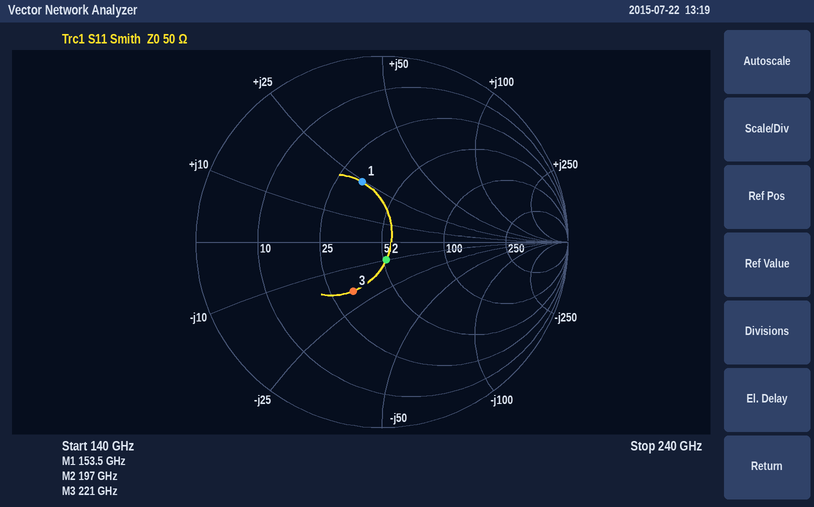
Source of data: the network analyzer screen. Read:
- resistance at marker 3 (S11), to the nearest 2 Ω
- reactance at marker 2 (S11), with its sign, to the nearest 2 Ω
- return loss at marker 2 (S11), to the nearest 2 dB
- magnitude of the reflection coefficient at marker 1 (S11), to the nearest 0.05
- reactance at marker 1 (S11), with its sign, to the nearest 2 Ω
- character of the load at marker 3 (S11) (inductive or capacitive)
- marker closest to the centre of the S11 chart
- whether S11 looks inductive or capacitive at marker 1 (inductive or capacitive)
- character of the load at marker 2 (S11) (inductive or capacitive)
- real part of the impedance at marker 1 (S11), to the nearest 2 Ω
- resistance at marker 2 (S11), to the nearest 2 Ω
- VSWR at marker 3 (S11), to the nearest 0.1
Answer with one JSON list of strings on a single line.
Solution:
["32 Ω", "-10 Ω", "20 dB", "0.35", "+24 Ω", "capacitive", "marker 2", "inductive", "capacitive", "34 Ω", "52 Ω", "1.9"]
